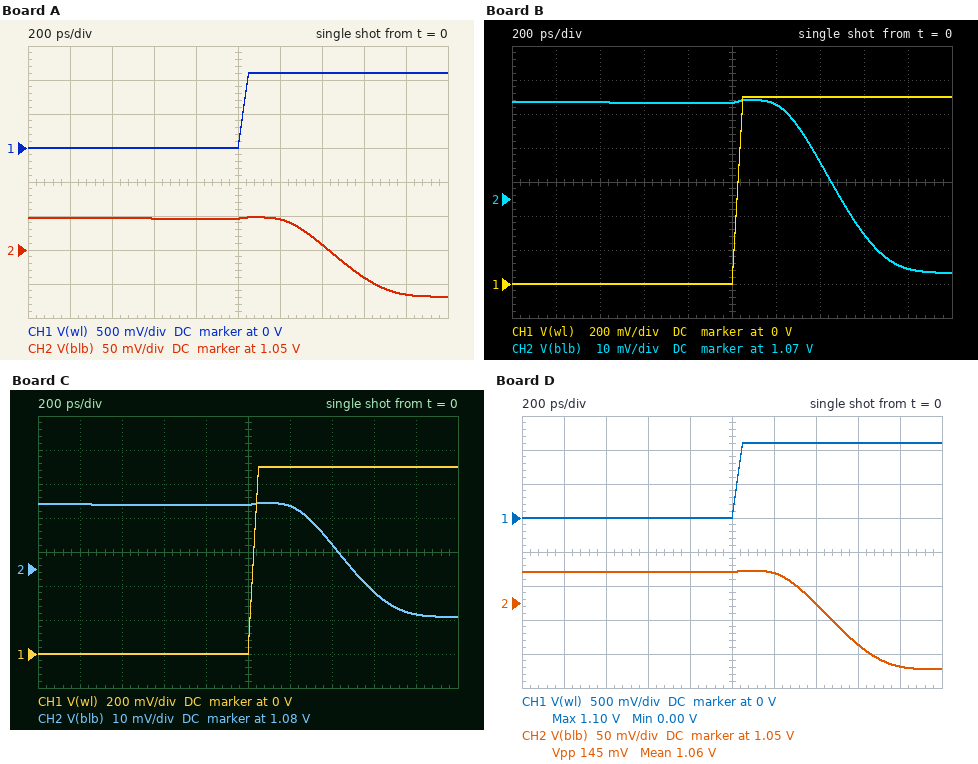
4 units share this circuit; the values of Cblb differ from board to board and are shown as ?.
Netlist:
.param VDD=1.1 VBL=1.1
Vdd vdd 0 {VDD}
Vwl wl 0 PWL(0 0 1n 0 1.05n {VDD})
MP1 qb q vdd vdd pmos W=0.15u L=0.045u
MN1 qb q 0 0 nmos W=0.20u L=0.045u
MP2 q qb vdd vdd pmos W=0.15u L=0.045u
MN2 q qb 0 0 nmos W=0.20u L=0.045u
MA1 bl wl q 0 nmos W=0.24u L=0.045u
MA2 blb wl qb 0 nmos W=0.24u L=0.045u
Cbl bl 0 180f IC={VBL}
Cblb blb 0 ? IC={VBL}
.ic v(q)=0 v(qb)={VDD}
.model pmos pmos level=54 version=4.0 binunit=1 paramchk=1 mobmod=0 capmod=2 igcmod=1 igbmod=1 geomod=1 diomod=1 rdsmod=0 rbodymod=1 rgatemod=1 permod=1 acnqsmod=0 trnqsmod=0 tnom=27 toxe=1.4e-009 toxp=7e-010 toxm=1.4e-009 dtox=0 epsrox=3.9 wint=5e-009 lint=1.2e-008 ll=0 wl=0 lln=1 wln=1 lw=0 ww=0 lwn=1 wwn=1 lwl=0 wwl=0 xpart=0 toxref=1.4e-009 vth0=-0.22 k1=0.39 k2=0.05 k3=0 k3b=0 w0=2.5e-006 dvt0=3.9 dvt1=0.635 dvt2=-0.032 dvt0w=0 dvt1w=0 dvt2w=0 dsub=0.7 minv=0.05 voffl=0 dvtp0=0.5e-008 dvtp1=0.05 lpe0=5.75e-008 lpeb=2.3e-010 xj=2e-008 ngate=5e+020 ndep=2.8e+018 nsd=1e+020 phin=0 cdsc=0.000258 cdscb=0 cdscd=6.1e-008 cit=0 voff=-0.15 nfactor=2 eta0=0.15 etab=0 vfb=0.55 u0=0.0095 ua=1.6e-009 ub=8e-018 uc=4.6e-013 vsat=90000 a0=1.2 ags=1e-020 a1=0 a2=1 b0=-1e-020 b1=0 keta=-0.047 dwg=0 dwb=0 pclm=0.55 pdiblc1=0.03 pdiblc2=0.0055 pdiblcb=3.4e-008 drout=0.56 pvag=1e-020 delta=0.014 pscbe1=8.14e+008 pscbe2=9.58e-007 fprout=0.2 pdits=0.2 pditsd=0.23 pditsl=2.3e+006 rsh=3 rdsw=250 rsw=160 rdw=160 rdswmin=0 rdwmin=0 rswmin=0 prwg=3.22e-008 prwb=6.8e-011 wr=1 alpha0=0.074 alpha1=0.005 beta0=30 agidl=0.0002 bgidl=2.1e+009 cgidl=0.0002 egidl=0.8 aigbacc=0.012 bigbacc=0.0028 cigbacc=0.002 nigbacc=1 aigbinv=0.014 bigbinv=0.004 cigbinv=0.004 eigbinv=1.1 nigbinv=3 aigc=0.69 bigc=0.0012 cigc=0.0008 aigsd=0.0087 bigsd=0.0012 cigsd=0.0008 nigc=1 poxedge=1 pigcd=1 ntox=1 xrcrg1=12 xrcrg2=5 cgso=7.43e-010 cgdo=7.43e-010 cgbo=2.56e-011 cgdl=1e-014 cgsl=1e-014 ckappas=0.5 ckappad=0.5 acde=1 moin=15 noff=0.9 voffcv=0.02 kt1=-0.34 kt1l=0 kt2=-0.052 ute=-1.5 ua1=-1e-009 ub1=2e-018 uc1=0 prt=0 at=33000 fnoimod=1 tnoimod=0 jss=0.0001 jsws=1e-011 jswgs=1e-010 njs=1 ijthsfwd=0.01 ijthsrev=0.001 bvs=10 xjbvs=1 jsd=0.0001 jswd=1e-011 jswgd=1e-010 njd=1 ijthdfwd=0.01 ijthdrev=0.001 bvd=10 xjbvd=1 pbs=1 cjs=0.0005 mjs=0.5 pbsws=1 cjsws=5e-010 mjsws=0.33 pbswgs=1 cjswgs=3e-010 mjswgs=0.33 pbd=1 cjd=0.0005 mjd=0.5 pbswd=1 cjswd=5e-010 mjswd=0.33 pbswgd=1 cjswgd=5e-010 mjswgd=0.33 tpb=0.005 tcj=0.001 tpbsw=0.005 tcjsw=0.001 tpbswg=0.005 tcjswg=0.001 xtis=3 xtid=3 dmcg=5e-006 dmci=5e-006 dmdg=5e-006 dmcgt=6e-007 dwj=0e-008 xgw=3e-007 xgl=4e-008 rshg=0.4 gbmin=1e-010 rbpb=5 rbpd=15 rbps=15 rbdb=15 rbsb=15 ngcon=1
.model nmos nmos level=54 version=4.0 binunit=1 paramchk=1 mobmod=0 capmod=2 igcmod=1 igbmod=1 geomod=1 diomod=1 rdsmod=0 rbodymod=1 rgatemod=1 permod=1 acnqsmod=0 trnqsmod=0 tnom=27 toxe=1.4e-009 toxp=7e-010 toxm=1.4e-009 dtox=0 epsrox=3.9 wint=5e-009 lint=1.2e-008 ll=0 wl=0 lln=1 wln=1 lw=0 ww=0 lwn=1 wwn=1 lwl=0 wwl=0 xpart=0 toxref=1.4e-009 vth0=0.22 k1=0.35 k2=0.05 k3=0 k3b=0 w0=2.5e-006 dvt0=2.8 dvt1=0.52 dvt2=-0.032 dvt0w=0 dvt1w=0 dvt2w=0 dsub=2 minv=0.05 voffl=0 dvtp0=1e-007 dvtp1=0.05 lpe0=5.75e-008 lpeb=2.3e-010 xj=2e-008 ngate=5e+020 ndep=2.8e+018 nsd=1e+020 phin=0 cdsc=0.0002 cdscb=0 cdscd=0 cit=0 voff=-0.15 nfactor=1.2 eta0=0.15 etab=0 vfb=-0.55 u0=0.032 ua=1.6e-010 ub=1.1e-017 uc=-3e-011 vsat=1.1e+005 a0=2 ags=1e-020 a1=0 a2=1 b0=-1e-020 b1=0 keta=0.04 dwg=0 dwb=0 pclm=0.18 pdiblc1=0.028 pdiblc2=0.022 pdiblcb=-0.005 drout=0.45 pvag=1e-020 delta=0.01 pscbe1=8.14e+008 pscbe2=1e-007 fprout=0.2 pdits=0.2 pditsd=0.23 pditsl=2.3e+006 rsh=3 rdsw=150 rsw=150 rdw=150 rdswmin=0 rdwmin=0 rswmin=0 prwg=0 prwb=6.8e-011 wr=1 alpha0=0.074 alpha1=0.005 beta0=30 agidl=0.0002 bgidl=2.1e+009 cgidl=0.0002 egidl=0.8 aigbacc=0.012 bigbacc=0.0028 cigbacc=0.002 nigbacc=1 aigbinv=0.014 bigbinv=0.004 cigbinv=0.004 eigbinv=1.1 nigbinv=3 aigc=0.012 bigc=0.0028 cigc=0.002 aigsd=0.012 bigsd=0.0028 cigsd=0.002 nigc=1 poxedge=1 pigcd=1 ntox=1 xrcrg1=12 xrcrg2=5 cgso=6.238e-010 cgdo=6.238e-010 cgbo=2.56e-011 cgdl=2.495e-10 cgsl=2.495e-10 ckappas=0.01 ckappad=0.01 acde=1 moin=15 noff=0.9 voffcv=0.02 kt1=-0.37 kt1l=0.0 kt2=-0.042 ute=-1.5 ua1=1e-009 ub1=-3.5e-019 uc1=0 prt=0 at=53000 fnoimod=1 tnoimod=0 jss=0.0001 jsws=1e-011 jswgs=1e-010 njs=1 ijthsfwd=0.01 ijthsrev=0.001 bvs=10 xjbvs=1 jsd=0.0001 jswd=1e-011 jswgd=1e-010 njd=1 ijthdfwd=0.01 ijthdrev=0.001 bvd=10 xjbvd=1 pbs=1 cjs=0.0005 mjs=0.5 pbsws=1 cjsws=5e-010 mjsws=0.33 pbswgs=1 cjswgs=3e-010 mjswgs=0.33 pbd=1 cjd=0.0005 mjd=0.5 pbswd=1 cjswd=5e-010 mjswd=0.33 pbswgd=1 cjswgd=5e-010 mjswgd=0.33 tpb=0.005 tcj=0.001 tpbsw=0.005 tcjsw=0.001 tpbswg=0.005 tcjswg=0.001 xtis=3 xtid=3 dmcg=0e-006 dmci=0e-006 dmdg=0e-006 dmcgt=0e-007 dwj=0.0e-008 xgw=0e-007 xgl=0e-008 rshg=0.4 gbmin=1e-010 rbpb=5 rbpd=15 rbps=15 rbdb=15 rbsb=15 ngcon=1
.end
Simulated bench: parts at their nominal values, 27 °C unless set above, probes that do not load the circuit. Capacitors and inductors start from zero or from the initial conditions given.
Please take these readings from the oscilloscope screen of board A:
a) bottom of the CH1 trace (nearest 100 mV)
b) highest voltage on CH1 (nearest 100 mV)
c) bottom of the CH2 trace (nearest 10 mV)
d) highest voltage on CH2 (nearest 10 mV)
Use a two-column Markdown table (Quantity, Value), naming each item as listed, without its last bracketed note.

| Quantity | Value |
|---|---|
| bottom of the CH1 trace | 0 V |
| highest voltage on CH1 | 1.1 V |
| bottom of the CH2 trace | 980 mV |
| highest voltage on CH2 | 1.10 V |
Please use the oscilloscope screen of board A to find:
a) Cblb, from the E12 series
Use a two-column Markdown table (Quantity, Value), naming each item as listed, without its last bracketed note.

| Quantity | Value |
|---|---|
| Cblb, from the E12 series | 100 fF |
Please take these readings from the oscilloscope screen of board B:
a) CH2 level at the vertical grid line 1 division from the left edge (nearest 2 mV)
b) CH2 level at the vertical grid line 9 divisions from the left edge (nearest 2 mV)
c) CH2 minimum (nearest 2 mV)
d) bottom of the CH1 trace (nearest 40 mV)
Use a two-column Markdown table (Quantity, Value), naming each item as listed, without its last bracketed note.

| Quantity | Value |
|---|---|
| CH2 level at the vertical grid line 1 division from the left edge | 1.098 V |
| CH2 level at the vertical grid line 9 divisions from the left edge | 1.050 V |
| CH2 minimum | 1.048 V |
| bottom of the CH1 trace | 0 V |
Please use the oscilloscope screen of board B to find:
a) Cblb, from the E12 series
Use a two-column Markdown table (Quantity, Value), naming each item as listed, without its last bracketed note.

| Quantity | Value |
|---|---|
| Cblb, from the E12 series | 220 fF |
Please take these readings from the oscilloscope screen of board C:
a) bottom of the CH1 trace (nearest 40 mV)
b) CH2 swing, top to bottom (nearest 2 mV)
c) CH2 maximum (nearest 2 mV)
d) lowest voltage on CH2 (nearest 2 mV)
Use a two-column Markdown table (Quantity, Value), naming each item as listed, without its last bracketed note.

| Quantity | Value |
|---|---|
| bottom of the CH1 trace | 0 V |
| CH2 swing, top to bottom | 34 mV |
| CH2 maximum | 1.100 V |
| lowest voltage on CH2 | 1.066 V |
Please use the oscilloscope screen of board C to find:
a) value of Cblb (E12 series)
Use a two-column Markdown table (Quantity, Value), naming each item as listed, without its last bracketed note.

| Quantity | Value |
|---|---|
| value of Cblb | 330 fF |
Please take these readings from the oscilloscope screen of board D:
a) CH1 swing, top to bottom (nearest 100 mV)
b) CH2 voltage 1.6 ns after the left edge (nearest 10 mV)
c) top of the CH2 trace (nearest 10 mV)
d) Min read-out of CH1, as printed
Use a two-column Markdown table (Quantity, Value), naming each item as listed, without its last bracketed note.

| Quantity | Value |
|---|---|
| CH1 swing, top to bottom | 1.1 V |
| CH2 voltage 1.6 ns after the left edge | 990 mV |
| top of the CH2 trace | 1.10 V |
| Min read-out of CH1, as printed | 0.00 V |
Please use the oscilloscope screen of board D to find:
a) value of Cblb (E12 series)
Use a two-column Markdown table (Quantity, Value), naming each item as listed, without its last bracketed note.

| Quantity | Value |
|---|---|
| value of Cblb | 82 fF |
